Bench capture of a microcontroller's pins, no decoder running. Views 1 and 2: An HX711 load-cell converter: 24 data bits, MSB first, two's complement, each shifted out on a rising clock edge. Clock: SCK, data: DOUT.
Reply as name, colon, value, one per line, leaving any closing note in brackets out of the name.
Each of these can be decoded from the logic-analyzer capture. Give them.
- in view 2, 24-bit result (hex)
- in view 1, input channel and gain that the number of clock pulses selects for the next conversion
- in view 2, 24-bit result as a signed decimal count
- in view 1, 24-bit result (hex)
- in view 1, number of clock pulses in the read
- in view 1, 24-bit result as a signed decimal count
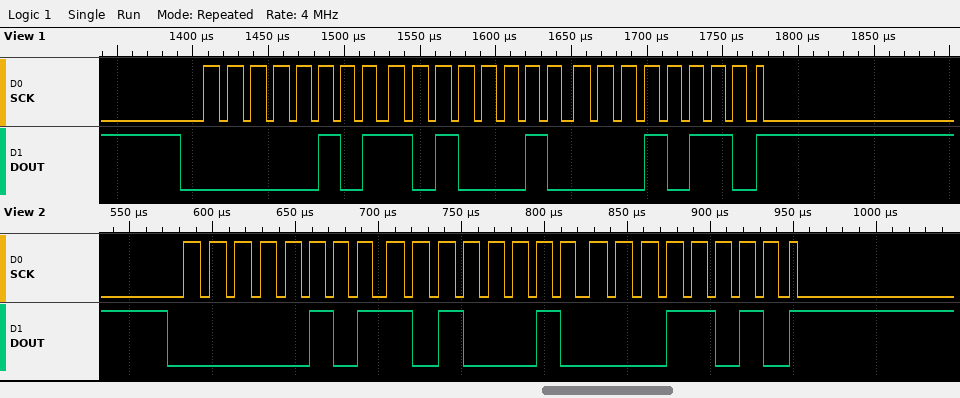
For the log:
in view 2, 24-bit result: 0x05A21A
in view 1, input channel and gain that the number of clock pulses selects for the next conversion: channel A, gain 128
in view 2, 24-bit result as a signed decimal count: 369178
in view 1, 24-bit result: 0x05A216
in view 1, number of clock pulses in the read: 25
in view 1, 24-bit result as a signed decimal count: 369174
